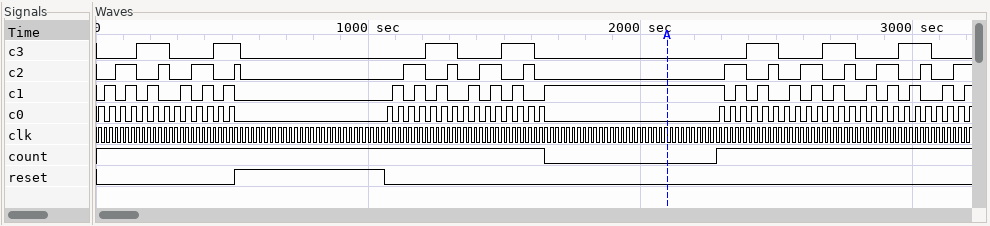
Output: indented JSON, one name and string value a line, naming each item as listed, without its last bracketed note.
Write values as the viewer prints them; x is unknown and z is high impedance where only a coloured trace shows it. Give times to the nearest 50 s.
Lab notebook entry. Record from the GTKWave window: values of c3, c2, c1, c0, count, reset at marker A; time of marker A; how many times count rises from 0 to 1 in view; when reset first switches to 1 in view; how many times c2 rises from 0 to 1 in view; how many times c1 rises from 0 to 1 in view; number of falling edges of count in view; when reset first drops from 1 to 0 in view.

{
  "values of c3, c2, c1, c0, count, reset at marker A": "c3=0, c2=0, c1=1, c0=0, count=0, reset=0",
  "time of marker A": "2100 s",
  "how many times count rises from 0 to 1 in view": "1",
  "when reset first switches to 1 in view": "500 s",
  "how many times c2 rises from 0 to 1 in view": "15",
  "how many times c1 rises from 0 to 1 in view": "23",
  "number of falling edges of count in view": "1",
  "when reset first drops from 1 to 0 in view": "1050 s"
}
